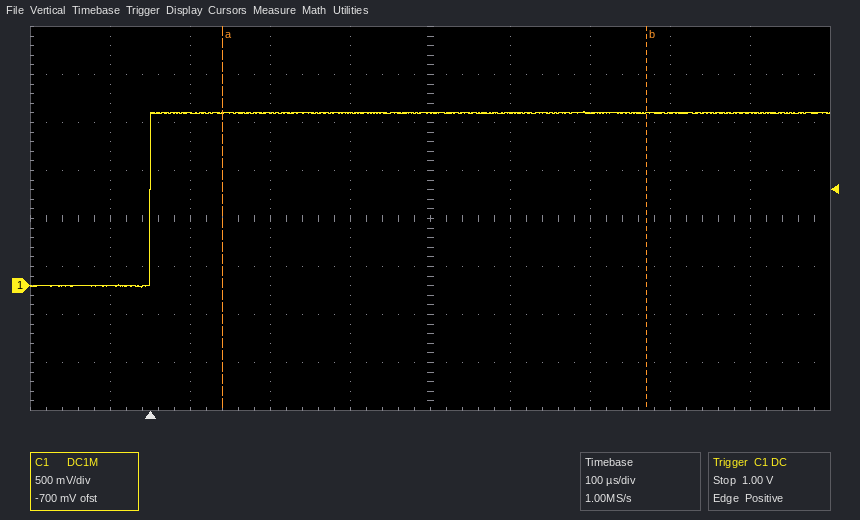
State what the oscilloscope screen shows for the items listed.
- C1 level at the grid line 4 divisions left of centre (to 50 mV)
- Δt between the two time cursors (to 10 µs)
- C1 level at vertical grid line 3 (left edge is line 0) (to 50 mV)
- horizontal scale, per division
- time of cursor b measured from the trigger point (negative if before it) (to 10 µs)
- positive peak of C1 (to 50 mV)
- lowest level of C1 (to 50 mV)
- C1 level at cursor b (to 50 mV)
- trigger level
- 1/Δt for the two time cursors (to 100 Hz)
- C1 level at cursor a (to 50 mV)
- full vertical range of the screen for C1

0 mV
530 µs
1.80 V
100 µs
+620 µs
1.80 V
0 mV
1.80 V
1.00 V
1.9 kHz
1.80 V
4 V
